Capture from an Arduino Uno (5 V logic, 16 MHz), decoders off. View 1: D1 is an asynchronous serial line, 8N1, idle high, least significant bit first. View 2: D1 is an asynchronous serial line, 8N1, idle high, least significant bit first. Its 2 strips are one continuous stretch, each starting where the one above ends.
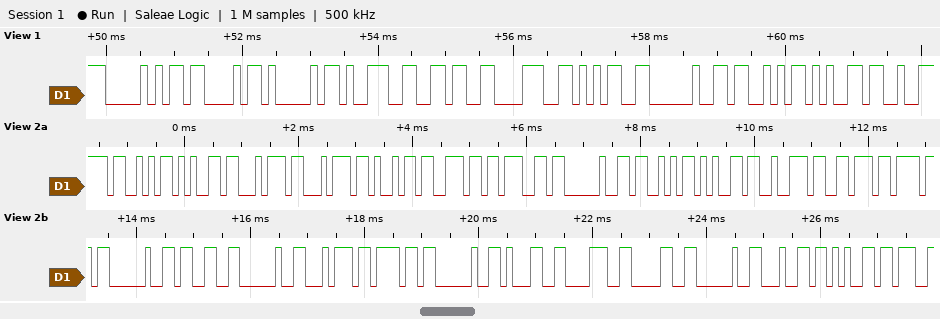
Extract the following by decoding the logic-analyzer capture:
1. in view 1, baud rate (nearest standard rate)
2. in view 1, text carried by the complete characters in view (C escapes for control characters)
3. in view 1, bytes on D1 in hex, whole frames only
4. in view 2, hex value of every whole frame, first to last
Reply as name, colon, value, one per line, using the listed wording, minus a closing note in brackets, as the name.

in view 1, baud rate: 9600 baud
in view 1, text carried by the complete characters in view: "PCA9685 Se"
in view 1, bytes on D1 in hex, whole frames only: 50 43 41 39 36 38 35 20 53 65
in view 2, hex value of every whole frame, first to last: 53 65 74 74 69 6E 67 20 53 65 72 76 6F 20 33 20 74 6F 20 31 38 30 20 64 65
